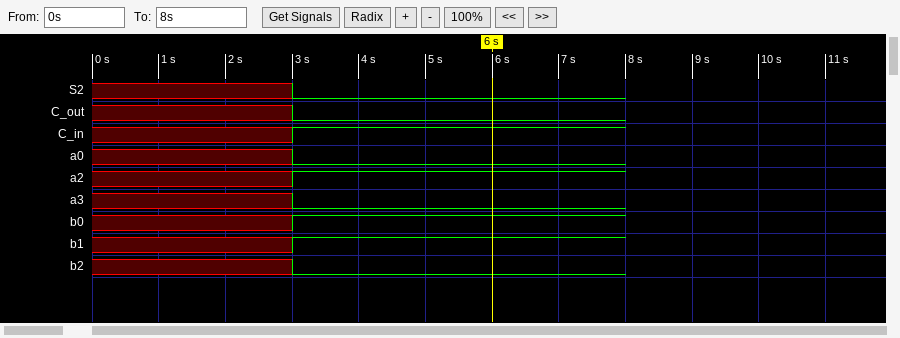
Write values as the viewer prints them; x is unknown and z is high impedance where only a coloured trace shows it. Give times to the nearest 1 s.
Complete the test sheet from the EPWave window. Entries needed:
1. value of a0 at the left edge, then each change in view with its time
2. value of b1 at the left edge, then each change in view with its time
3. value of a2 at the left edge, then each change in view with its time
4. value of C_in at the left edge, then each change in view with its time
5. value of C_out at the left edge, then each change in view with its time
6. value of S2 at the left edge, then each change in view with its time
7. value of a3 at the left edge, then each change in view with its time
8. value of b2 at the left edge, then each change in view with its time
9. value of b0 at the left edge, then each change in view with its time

x, 0 at 3 s
x, 1 at 3 s
x, 1 at 3 s
x, 1 at 3 s
x, 0 at 3 s
x, 0 at 3 s
x, 0 at 3 s
x, 0 at 3 s
x, 1 at 3 s
